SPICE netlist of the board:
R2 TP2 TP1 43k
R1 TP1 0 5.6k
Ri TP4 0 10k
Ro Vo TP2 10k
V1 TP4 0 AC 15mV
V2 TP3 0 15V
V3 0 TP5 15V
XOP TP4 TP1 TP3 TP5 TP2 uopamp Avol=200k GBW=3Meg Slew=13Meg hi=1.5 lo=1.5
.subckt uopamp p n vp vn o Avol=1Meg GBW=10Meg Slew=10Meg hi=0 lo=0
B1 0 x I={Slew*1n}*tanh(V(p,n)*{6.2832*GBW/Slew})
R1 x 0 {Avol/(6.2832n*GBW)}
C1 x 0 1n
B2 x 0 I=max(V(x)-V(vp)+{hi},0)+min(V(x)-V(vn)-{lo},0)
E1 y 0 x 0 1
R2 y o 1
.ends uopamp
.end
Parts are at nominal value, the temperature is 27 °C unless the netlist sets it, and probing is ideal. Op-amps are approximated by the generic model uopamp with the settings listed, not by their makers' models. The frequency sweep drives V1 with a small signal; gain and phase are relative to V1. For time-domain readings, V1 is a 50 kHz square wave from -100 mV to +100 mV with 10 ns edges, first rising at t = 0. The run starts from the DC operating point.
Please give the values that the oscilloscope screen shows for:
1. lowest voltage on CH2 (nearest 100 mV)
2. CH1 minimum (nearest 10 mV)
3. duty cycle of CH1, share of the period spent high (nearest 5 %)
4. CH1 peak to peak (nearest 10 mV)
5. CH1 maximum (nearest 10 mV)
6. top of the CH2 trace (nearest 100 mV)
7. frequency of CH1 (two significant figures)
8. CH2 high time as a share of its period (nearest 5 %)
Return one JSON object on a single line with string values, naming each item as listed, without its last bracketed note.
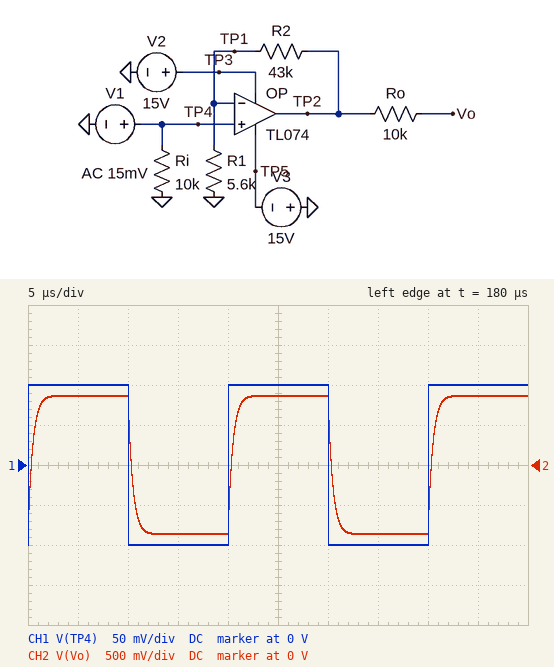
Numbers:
{"lowest voltage on CH2": "-900 mV", "CH1 minimum": "-100 mV", "duty cycle of CH1, share of the period spent high": "50 %", "CH1 peak to peak": "200 mV", "CH1 maximum": "100 mV", "top of the CH2 trace": "900 mV", "frequency of CH1": "50 kHz", "CH2 high time as a share of its period": "50 %"}
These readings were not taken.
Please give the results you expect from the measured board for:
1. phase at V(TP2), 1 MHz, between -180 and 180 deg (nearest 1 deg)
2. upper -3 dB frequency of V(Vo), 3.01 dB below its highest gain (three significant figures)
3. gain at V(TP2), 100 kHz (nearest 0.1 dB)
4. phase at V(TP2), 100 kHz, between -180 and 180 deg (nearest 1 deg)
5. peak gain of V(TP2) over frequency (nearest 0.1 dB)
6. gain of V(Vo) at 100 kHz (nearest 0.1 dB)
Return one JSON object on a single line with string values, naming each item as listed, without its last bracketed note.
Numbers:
{"phase at V(TP2), 1 MHz, between -180 and 180 deg": "-71 deg", "upper -3 dB frequency of V(Vo), 3.01 dB below its highest gain": "346 kHz", "gain at V(TP2), 100 kHz": "18.4 dB", "phase at V(TP2), 100 kHz, between -180 and 180 deg": "-16 deg", "peak gain of V(TP2) over frequency": "18.8 dB", "gain of V(Vo) at 100 kHz": "18.4 dB"}
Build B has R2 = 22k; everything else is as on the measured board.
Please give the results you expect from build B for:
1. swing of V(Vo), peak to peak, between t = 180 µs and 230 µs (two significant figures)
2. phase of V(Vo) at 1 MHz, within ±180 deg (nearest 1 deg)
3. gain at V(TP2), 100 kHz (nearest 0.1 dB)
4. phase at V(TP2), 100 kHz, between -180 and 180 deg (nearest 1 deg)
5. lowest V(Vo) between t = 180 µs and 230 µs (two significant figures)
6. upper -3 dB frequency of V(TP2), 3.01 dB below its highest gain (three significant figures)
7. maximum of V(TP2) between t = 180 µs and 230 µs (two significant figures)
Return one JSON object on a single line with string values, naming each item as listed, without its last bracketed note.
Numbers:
{"swing of V(Vo), peak to peak, between t = 180 µs and 230 µs": "990 mV", "phase of V(Vo) at 1 MHz, within ±180 deg": "-59 deg", "gain at V(TP2), 100 kHz": "13.7 dB", "phase at V(TP2), 100 kHz, between -180 and 180 deg": "-9 deg", "lowest V(Vo) between t = 180 µs and 230 µs": "-490 mV", "upper -3 dB frequency of V(TP2), 3.01 dB below its highest gain": "609 kHz", "maximum of V(TP2) between t = 180 µs and 230 µs": "490 mV"}
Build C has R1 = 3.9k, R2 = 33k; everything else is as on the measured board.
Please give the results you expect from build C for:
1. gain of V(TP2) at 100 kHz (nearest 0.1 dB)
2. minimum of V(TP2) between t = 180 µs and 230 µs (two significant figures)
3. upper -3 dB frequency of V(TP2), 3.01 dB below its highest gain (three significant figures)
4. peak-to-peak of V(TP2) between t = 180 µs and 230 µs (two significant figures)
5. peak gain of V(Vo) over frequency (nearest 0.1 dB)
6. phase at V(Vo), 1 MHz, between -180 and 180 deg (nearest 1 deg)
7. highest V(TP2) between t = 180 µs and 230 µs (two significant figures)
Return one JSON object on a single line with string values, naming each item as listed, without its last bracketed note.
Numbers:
{"gain of V(TP2) at 100 kHz": "19.1 dB", "minimum of V(TP2) between t = 180 µs and 230 µs": "-950 mV", "upper -3 dB frequency of V(TP2), 3.01 dB below its highest gain": "317 kHz", "peak-to-peak of V(TP2) between t = 180 µs and 230 µs": "1.9 V", "peak gain of V(Vo) over frequency": "19.5 dB", "phase at V(Vo), 1 MHz, between -180 and 180 deg": "-72 deg", "highest V(TP2) between t = 180 µs and 230 µs": "950 mV"}
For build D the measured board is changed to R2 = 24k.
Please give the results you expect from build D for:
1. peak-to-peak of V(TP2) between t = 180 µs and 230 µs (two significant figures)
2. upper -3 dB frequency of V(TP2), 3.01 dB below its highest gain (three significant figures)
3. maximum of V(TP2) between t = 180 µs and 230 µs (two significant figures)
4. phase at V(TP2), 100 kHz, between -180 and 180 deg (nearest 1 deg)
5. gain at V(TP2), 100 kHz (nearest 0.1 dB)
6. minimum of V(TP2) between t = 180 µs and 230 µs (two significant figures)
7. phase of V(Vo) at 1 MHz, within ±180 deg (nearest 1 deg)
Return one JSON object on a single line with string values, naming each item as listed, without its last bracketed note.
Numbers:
{"peak-to-peak of V(TP2) between t = 180 µs and 230 µs": "1.1 V", "upper -3 dB frequency of V(TP2), 3.01 dB below its highest gain": "568 kHz", "maximum of V(TP2) between t = 180 µs and 230 µs": "530 mV", "phase at V(TP2), 100 kHz, between -180 and 180 deg": "-10 deg", "gain at V(TP2), 100 kHz": "14.3 dB", "minimum of V(TP2) between t = 180 µs and 230 µs": "-530 mV", "phase of V(Vo) at 1 MHz, within ±180 deg": "-60 deg"}
